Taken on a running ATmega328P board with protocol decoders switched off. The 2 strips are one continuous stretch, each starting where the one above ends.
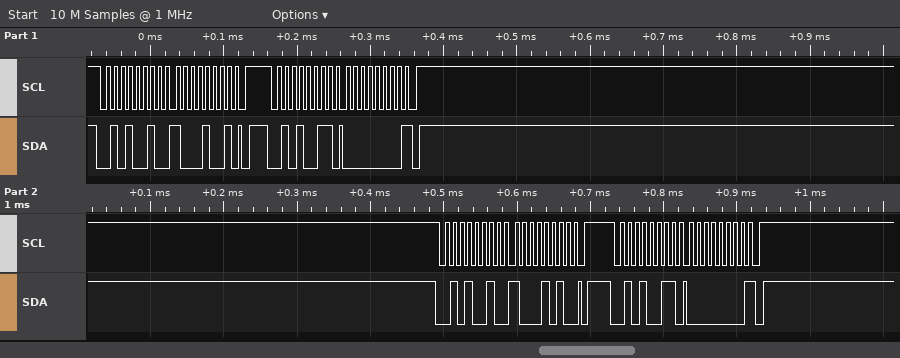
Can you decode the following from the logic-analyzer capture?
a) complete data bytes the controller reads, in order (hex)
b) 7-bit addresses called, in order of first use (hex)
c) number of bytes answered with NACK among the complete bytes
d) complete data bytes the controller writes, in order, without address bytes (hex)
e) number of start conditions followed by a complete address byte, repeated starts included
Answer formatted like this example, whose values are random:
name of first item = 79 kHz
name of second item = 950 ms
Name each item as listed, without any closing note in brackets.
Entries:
complete data bytes the controller reads, in order = 00 00
7-bit addresses called, in order of first use = 0x29
number of bytes answered with NACK among the complete bytes = 2
complete data bytes the controller writes, in order, without address bytes = 89 8A
number of start conditions followed by a complete address byte, repeated starts included = 4
